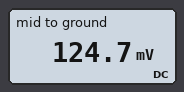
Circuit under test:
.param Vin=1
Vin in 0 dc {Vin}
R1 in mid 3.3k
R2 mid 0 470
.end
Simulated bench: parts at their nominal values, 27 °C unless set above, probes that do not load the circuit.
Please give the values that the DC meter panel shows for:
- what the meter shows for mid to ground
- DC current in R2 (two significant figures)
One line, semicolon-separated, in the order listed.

124.7 mV; 270 µA
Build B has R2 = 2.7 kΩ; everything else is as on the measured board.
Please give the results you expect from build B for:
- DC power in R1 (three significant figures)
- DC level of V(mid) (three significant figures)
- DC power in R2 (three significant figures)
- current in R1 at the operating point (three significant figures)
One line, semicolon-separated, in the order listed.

91.7 µW; 450 mV; 75.0 µW; 167 µA
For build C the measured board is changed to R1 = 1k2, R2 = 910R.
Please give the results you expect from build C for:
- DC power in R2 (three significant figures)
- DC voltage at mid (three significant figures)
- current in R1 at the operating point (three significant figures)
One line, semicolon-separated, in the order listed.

204 µW; 431 mV; 474 µA
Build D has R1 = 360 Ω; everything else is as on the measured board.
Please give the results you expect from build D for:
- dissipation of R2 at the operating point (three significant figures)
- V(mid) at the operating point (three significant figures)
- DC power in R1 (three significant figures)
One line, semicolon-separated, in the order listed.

682 µW; 566 mV; 523 µW
